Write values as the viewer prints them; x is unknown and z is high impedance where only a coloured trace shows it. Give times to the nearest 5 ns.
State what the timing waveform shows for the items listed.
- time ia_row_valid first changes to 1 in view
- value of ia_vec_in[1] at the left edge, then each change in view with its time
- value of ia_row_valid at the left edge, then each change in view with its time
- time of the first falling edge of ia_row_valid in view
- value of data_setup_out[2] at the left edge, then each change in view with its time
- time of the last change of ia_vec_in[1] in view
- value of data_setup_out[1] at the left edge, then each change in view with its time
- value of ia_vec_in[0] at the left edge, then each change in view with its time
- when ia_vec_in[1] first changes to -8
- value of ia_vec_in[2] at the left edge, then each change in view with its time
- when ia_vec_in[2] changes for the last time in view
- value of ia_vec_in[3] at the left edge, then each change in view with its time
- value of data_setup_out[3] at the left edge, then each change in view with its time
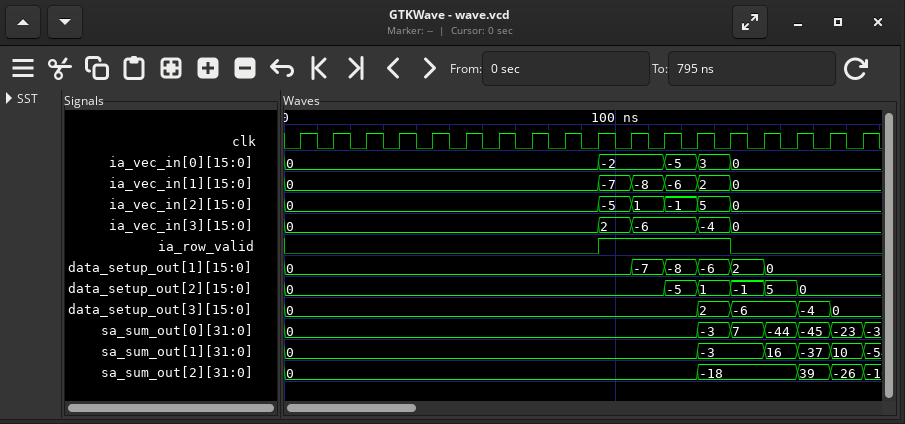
95 ns
0, -7 at 95 ns, -8 at 105 ns, -6 at 115 ns, 2 at 125 ns, 0 at 135 ns
0, 1 at 95 ns, 0 at 135 ns
135 ns
0, -5 at 115 ns, 1 at 125 ns, -1 at 135 ns, 5 at 145 ns, 0 at 155 ns
135 ns
0, -7 at 105 ns, -8 at 115 ns, -6 at 125 ns, 2 at 135 ns, 0 at 145 ns
0, -2 at 95 ns, -5 at 115 ns, 3 at 125 ns, 0 at 135 ns
105 ns
0, -5 at 95 ns, 1 at 105 ns, -1 at 115 ns, 5 at 125 ns, 0 at 135 ns
135 ns
0, 2 at 95 ns, -6 at 105 ns, -4 at 125 ns, 0 at 135 ns
0, 2 at 125 ns, -6 at 135 ns, -4 at 155 ns, 0 at 165 ns
